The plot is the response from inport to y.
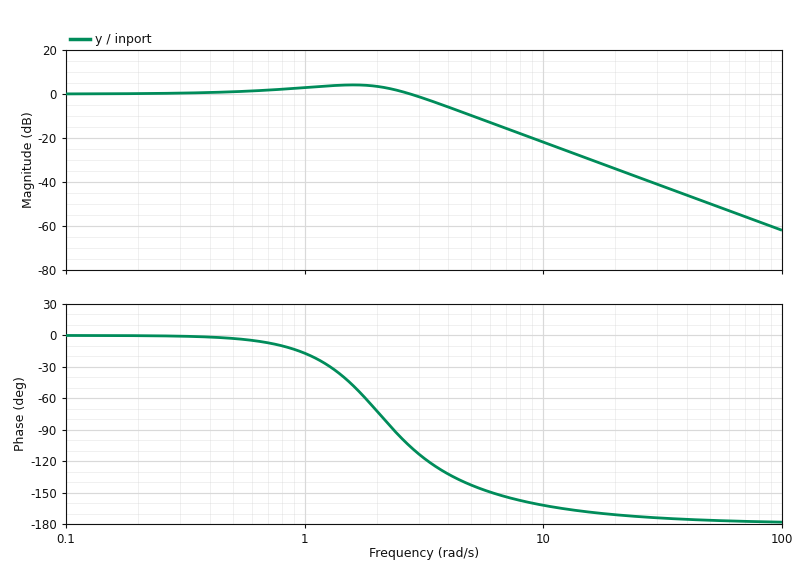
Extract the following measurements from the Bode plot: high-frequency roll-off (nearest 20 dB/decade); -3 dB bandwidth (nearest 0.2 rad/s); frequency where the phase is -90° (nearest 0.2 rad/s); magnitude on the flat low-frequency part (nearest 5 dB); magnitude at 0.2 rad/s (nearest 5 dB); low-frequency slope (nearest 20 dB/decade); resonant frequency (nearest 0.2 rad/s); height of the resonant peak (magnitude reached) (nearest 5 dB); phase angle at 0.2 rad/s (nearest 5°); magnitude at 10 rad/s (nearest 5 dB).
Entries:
-40 dB/decade
3.4 rad/s
2.4 rad/s
0 dB
0 dB
0 dB/decade
1.6 rad/s
5 dB
0°
-20 dB
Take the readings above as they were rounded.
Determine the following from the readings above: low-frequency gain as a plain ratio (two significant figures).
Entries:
1.0
